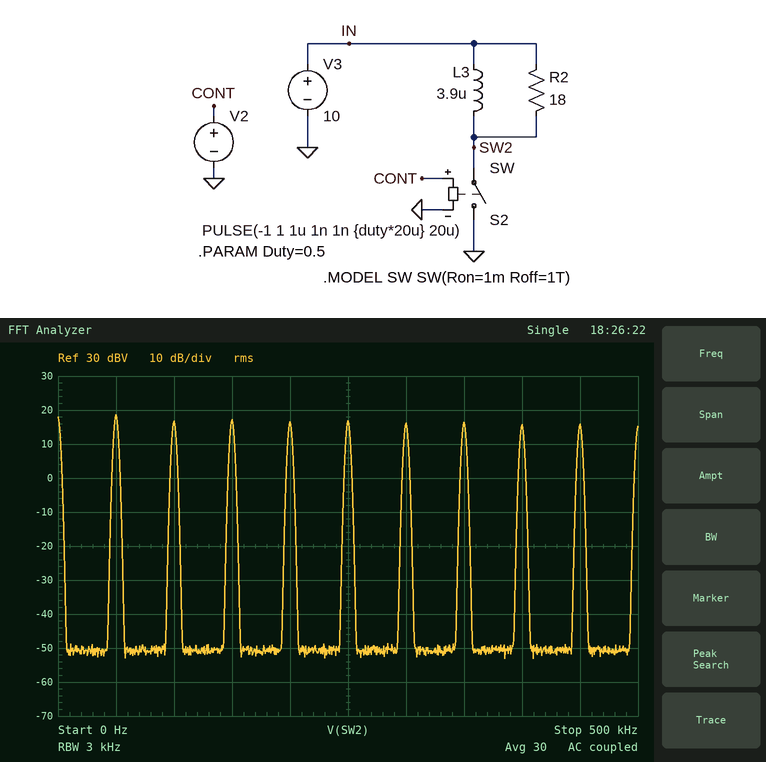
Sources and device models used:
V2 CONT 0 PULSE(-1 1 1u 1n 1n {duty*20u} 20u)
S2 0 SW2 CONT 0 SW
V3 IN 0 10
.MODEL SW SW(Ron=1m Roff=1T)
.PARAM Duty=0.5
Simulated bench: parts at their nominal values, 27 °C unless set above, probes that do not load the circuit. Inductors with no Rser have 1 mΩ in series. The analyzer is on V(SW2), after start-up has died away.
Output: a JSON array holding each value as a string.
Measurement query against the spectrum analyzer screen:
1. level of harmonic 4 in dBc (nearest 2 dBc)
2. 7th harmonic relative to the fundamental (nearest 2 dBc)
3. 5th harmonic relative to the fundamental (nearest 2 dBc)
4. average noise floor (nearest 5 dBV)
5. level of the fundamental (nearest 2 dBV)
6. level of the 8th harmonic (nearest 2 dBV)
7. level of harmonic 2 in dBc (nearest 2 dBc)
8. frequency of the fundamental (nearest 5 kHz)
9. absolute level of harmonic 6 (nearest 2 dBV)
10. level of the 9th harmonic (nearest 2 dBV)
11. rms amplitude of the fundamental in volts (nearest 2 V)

["-2 dBc", "-2 dBc", "-2 dBc", "-50 dBV", "18 dBV", "16 dBV", "-2 dBc", "50 kHz", "16 dBV", "16 dBV", "8 V"]
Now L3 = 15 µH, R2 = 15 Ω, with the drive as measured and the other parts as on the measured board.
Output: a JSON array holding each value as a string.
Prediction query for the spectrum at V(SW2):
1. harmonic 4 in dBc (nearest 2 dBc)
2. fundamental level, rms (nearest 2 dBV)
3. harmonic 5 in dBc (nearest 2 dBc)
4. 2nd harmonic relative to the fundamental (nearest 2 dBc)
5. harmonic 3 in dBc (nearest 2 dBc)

["-6 dBc", "20 dBV", "-6 dBc", "-4 dBc", "-4 dBc"]
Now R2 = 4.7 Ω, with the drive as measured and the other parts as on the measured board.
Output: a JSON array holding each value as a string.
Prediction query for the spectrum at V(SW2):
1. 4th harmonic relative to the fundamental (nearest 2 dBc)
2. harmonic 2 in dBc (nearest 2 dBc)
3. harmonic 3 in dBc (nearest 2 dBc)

["-6 dBc", "-4 dBc", "-2 dBc"]
